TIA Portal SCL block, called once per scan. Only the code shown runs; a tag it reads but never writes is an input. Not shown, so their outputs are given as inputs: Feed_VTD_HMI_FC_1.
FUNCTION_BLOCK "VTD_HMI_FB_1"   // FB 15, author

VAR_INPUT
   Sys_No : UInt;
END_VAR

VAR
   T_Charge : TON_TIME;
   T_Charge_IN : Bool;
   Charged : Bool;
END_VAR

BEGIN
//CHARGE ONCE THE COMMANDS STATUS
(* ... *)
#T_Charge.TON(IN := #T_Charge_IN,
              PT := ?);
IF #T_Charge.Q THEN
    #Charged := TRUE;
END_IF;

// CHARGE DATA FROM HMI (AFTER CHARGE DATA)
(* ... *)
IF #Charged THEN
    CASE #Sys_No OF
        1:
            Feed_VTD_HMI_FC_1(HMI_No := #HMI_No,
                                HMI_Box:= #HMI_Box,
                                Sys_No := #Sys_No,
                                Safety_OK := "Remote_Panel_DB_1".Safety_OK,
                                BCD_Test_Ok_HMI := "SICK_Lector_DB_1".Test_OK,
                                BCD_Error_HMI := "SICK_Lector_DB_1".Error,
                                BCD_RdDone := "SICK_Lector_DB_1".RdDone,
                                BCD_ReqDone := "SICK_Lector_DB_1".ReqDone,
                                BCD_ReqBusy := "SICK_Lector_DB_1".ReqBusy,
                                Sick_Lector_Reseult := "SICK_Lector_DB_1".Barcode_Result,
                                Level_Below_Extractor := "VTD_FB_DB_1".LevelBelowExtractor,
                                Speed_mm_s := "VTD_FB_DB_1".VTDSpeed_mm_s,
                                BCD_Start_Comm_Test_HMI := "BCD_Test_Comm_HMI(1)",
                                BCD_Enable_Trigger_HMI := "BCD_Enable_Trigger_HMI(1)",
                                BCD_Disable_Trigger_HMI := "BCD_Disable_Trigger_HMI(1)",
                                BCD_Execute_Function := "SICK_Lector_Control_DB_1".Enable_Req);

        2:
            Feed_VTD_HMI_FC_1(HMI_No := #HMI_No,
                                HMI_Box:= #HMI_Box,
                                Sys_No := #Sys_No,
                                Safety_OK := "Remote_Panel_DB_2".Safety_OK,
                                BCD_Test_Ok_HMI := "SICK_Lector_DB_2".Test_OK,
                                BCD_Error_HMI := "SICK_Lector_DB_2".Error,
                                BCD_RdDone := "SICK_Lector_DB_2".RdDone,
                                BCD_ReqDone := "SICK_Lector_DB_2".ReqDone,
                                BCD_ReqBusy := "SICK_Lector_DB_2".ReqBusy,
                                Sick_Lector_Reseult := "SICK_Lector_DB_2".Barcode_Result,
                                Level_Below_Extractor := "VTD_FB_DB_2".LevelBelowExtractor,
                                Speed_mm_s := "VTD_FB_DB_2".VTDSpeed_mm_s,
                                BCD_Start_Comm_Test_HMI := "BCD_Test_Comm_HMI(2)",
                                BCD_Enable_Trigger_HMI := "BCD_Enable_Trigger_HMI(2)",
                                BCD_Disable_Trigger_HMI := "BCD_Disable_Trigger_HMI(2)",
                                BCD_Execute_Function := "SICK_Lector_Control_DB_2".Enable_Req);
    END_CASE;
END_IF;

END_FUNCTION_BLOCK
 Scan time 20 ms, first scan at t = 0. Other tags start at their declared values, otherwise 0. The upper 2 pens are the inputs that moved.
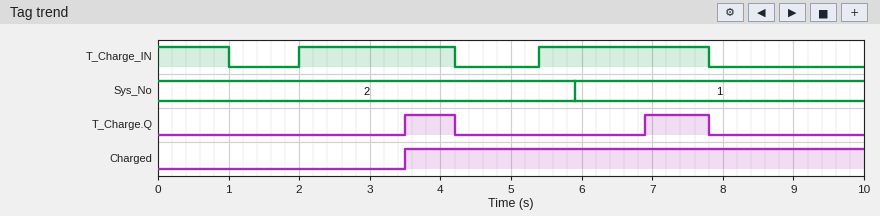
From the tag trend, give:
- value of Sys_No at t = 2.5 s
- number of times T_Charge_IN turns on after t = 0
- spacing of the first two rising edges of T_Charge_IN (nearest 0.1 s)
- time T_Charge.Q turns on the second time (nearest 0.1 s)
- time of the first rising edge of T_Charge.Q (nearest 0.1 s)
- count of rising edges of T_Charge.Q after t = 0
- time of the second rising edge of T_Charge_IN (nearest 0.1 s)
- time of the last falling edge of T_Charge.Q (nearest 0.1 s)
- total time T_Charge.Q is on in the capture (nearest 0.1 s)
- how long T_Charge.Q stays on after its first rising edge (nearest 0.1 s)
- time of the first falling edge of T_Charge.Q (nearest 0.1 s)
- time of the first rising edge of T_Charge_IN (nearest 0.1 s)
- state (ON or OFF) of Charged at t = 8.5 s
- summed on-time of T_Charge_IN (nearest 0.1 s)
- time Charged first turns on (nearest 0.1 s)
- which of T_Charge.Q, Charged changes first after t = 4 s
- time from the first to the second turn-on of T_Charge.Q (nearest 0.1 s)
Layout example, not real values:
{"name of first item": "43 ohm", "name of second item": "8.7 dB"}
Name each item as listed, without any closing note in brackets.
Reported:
{"value of Sys_No at t = 2.5 s": "2", "number of times T_Charge_IN turns on after t = 0": "2", "spacing of the first two rising edges of T_Charge_IN": "3.4 s", "time T_Charge.Q turns on the second time": "6.9 s", "time of the first rising edge of T_Charge.Q": "3.5 s", "count of rising edges of T_Charge.Q after t = 0": "2", "time of the second rising edge of T_Charge_IN": "5.4 s", "time of the last falling edge of T_Charge.Q": "7.8 s", "total time T_Charge.Q is on in the capture": "1.6 s", "how long T_Charge.Q stays on after its first rising edge": "0.7 s", "time of the first falling edge of T_Charge.Q": "4.2 s", "time of the first rising edge of T_Charge_IN": "2.0 s", "state (ON or OFF) of Charged at t = 8.5 s": "ON", "summed on-time of T_Charge_IN": "5.6 s", "time Charged first turns on": "3.5 s", "which of T_Charge.Q, Charged changes first after t = 4 s": "T_Charge.Q", "time from the first to the second turn-on of T_Charge.Q": "3.4 s"}
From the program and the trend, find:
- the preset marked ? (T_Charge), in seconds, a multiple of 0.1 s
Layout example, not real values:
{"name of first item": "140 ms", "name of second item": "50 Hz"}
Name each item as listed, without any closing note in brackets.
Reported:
{"the preset marked ? (T_Charge), in seconds, a multiple of 0.1 s": "1.5 s"}
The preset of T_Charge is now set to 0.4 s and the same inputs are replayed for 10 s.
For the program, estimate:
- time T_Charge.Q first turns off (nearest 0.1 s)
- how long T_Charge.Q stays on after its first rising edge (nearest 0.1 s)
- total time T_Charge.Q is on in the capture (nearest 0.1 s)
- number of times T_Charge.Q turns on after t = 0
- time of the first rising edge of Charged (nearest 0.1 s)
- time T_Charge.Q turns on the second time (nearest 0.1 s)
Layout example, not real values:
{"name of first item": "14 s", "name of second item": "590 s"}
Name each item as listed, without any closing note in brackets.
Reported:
{"time T_Charge.Q first turns off": "1.0 s", "how long T_Charge.Q stays on after its first rising edge": "0.6 s", "total time T_Charge.Q is on in the capture": "4.4 s", "number of times T_Charge.Q turns on after t = 0": "3", "time of the first rising edge of Charged": "0.4 s", "time T_Charge.Q turns on the second time": "2.4 s"}
